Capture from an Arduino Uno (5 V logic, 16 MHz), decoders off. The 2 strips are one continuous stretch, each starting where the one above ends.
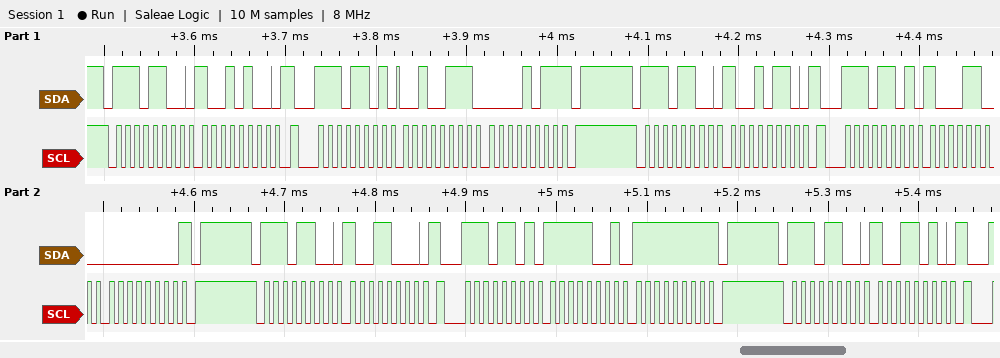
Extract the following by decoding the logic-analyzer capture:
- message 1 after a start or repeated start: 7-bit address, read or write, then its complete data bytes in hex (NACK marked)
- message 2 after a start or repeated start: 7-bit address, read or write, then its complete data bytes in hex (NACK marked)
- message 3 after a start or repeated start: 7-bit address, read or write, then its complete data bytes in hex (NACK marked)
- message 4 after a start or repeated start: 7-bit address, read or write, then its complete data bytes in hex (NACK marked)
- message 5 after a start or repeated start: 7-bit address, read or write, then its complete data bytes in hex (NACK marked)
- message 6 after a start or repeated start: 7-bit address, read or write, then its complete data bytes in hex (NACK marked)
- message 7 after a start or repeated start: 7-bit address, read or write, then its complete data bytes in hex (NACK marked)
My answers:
0x76 write: 94
0x76 read: 27 0B NACK
0x76 write: 96
0x76 read: 8C 00 NACK
0x76 write: 98
0x76 read: F9 FF NACK
0x76 write: 9A
